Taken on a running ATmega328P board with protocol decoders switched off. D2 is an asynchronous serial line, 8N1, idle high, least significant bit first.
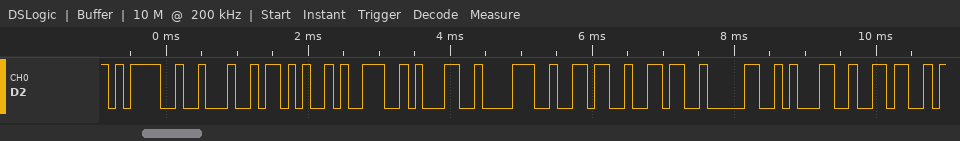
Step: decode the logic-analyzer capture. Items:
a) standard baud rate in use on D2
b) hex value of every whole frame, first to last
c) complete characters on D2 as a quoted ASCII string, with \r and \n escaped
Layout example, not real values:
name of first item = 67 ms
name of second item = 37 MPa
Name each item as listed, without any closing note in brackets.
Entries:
standard baud rate in use on D2 = 9600 baud
hex value of every whole frame, first to last = 0x3D 0x22 0x2B 0x39 0x31 0x38 0x36 0x36 0x30 0x31 0x36
complete characters on D2 as a quoted ASCII string, with \r and \n escaped = "=\"+91866016"
